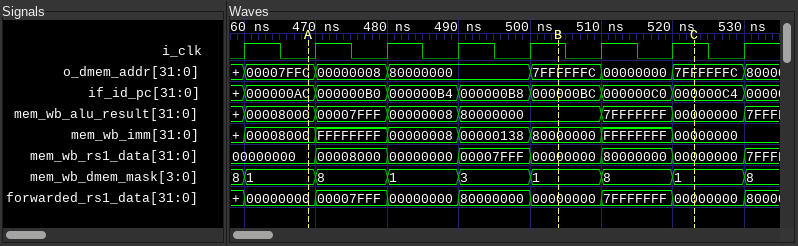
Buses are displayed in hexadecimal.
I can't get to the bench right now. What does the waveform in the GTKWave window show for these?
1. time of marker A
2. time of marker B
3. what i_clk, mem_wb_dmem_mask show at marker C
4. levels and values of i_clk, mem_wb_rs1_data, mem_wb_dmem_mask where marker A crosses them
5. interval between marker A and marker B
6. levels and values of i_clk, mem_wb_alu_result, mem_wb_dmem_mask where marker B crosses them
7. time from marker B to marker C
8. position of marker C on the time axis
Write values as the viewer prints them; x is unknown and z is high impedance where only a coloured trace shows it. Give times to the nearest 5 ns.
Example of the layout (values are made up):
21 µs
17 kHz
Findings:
470 ns
505 ns
i_clk=1, mem_wb_dmem_mask=1
i_clk=0, mem_wb_rs1_data=00000000, mem_wb_dmem_mask=1
35 ns
i_clk=1, mem_wb_alu_result=80000000, mem_wb_dmem_mask=1
20 ns
525 ns
